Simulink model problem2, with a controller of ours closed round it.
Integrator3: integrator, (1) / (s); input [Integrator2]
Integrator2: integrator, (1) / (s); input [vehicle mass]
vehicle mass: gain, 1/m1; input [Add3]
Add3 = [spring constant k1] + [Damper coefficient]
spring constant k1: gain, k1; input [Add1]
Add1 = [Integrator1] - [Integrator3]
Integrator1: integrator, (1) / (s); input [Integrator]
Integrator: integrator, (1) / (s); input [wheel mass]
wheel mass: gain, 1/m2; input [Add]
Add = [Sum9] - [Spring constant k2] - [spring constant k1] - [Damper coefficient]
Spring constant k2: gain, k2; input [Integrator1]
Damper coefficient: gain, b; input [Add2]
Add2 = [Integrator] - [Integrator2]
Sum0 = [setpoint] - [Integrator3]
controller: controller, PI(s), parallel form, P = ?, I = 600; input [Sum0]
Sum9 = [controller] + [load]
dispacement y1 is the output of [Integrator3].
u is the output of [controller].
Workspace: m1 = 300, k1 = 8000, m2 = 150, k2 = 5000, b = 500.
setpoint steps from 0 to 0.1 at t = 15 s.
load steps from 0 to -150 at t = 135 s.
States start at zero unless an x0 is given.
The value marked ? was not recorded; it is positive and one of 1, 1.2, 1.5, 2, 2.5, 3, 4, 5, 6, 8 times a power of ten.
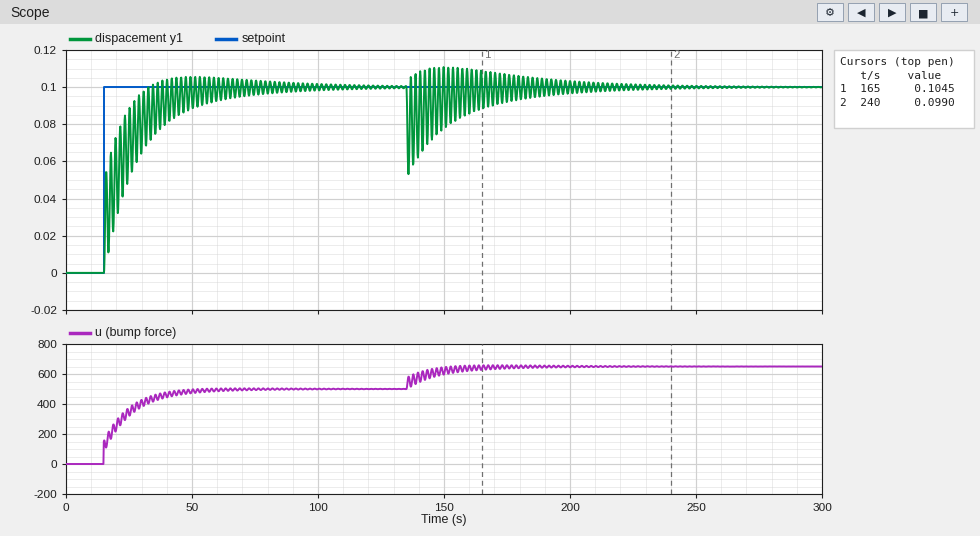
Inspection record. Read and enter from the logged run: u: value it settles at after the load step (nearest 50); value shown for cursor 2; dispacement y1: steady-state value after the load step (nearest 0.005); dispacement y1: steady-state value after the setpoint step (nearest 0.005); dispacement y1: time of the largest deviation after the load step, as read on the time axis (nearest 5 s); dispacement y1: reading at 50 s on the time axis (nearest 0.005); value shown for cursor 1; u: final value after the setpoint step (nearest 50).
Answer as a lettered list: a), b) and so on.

a) 650
b) 0.0990
c) 0.100
d) 0.100
e) 135 s
f) 0.095
g) 0.1045
h) 500
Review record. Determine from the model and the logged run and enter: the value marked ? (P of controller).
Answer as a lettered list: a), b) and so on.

a) 1500
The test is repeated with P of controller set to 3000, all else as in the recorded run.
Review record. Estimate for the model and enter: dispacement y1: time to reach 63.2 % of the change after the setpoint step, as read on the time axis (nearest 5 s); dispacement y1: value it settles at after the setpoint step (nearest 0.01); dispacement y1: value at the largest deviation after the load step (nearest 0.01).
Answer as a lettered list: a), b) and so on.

a) 15 s
b) 0.10
c) 0.06
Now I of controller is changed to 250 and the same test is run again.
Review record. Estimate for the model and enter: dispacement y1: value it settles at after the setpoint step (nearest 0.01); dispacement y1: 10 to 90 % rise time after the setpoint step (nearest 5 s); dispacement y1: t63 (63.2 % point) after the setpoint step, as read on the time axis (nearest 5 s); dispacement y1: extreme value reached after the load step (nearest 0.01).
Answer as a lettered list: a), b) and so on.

a) 0.10
b) 50 s
c) 25 s
d) 0.05
